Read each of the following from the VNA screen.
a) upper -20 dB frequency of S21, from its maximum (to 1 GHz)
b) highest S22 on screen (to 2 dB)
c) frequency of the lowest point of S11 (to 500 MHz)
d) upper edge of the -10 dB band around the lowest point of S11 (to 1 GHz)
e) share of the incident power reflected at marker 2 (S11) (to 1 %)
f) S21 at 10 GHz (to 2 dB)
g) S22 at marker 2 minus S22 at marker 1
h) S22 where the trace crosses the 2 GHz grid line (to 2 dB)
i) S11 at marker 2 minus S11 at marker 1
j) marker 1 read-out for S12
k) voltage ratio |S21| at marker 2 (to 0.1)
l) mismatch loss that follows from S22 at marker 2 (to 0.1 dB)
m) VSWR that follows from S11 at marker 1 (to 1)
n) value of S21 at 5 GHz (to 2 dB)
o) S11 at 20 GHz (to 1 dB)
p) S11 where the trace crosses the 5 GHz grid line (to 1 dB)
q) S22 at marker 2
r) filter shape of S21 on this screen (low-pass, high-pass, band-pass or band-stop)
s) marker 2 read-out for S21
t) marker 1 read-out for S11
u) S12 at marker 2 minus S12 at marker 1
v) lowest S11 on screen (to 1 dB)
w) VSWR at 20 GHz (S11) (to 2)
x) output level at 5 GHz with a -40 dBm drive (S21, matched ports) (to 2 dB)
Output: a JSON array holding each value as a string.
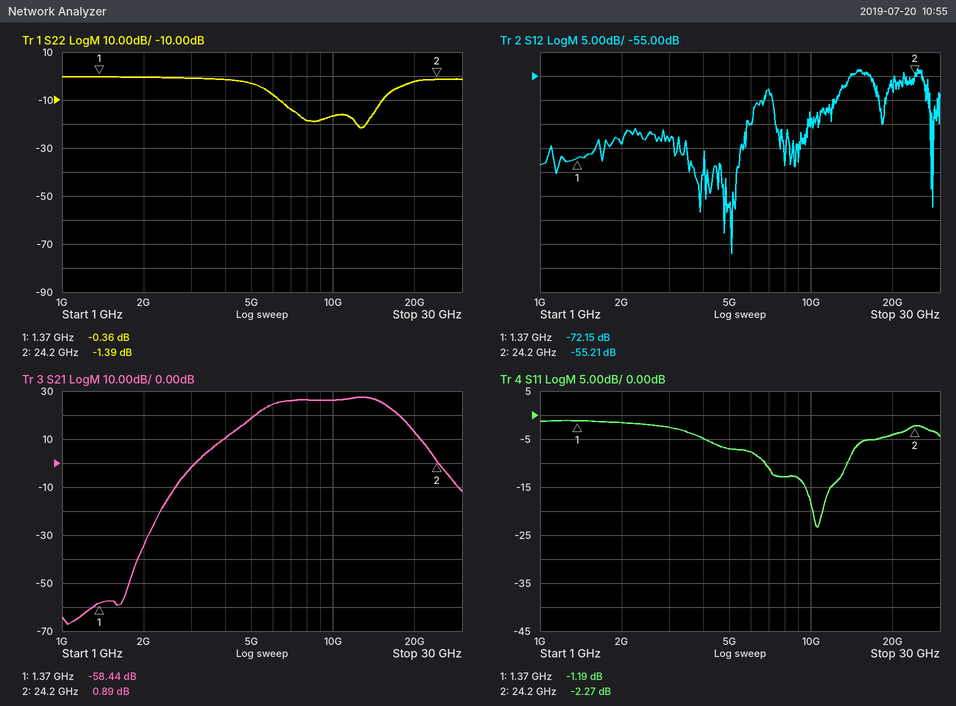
["22 GHz", "0 dB", "10.5 GHz", "14 GHz", "59 %", "26 dB", "-1.03 dB", "0 dB", "-1.08 dB", "-72.15 dB", "1.1", "5.6 dB", "15", "18 dB", "-4 dB", "-7 dB", "-1.39 dB", "band-pass", "0.89 dB", "-1.19 dB", "16.94 dB", "-23 dB", "4", "-22 dBm"]
